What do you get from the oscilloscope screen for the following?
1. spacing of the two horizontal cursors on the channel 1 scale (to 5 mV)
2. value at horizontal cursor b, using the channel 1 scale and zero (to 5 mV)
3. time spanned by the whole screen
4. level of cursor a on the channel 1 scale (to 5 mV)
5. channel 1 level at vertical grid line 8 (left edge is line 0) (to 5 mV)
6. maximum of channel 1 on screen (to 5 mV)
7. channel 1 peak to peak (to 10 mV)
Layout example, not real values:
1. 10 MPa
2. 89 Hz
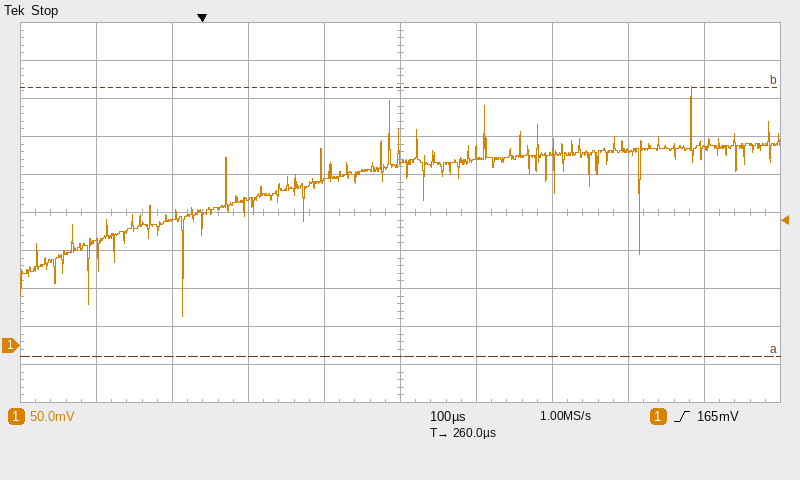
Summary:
1. 355 mV
2. 340 mV
3. 1 ms
4. -15 mV
5. 255 mV
6. 340 mV
7. 300 mV
